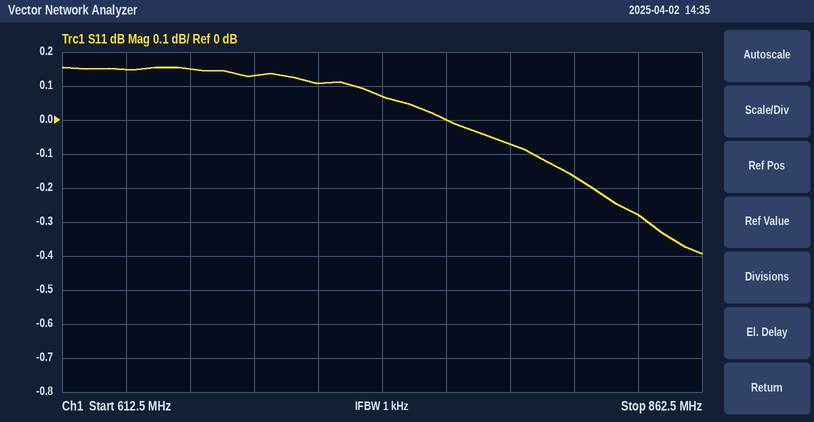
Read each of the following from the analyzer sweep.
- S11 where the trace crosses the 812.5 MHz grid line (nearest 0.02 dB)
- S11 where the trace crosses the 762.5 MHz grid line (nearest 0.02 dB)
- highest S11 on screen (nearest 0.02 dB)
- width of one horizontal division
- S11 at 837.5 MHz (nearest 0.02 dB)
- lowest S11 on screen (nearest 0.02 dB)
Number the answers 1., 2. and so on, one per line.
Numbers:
1. -0.16 dB
2. 0.00 dB
3. 0.16 dB
4. 25 MHz
5. -0.28 dB
6. -0.40 dB
